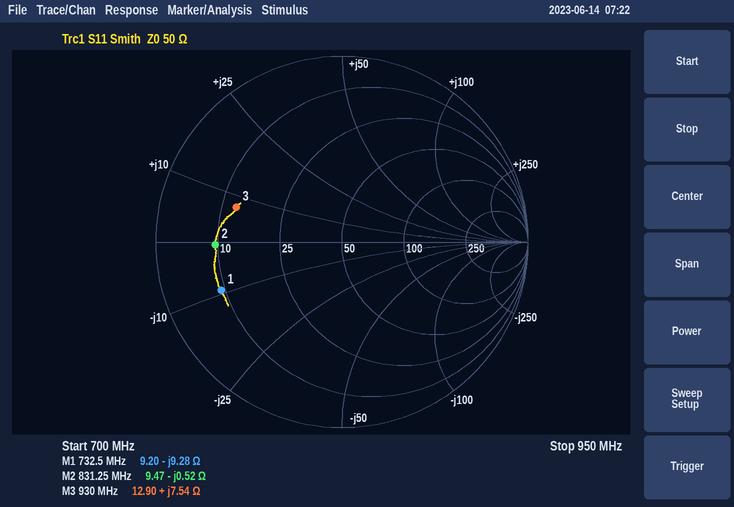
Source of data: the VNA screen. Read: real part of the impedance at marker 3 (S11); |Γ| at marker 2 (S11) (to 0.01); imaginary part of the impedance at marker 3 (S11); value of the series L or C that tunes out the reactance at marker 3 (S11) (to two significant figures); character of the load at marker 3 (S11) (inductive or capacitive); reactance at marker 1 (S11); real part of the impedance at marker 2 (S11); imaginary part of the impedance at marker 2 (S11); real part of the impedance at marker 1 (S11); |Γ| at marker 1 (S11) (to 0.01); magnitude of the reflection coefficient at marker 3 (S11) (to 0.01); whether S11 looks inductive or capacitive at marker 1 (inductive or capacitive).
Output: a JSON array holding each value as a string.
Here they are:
["12.90 Ω", "0.68", "+7.54 Ω", "23 pF", "inductive", "-9.28 Ω", "9.47 Ω", "-0.52 Ω", "9.20 Ω", "0.70", "0.60", "capacitive"]
